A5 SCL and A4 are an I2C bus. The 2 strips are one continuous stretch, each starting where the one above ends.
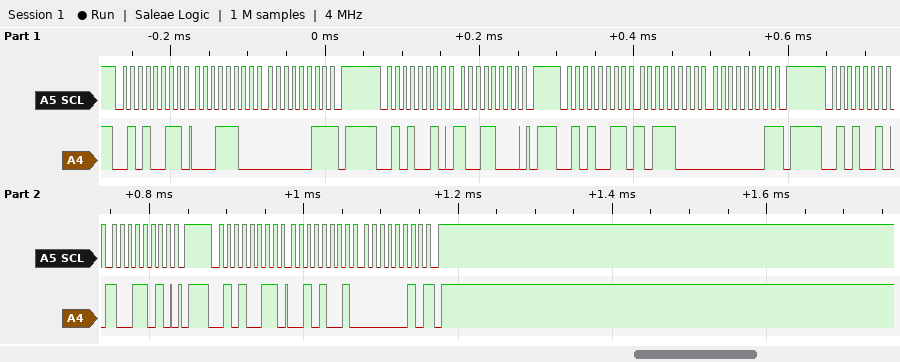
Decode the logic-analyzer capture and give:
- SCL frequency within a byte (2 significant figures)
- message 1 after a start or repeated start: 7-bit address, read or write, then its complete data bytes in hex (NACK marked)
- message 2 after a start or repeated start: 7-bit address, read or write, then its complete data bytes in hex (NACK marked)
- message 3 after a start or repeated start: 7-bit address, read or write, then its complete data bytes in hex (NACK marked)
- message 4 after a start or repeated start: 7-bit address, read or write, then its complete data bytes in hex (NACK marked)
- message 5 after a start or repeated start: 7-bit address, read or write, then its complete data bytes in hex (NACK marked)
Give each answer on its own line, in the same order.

100 kHz
0x29 read: 1C 03 NACK
0x29 write: 98
0x29 read: B8 01 NACK
0x29 write: 9A
0x29 read: 29 02 NACK
